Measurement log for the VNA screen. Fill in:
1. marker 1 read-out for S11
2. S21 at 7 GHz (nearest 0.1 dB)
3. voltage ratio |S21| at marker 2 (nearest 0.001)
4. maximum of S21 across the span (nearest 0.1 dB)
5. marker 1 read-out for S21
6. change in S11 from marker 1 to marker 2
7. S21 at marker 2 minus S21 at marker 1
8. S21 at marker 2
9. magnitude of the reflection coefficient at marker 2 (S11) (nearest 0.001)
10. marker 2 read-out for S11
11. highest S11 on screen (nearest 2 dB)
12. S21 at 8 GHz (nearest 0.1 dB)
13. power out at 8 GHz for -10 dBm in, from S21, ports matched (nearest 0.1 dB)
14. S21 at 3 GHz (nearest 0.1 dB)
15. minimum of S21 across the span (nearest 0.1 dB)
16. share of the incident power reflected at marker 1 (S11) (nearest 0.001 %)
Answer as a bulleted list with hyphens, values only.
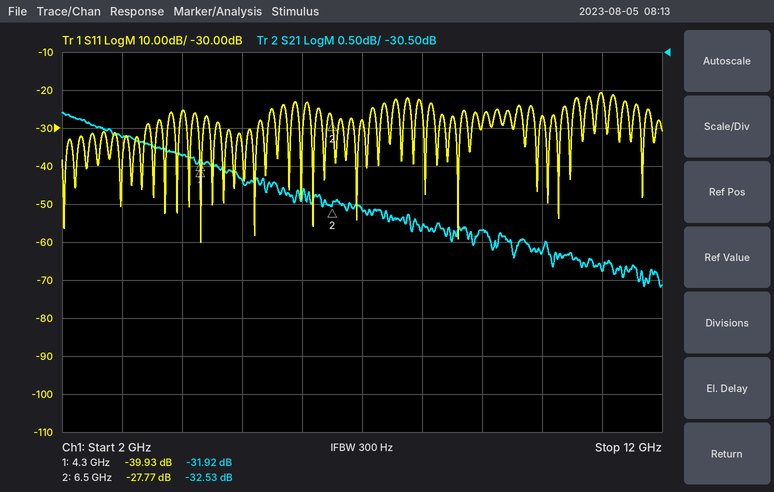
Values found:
- -39.93 dB
- -32.6 dB
- 0.024
- -31.3 dB
- -31.92 dB
- 12.16 dB
- -0.61 dB
- -32.53 dB
- 0.041
- -27.77 dB
- -20 dB
- -32.8 dB
- -42.8 dBm
- -31.6 dB
- -33.6 dB
- 0.010 %
